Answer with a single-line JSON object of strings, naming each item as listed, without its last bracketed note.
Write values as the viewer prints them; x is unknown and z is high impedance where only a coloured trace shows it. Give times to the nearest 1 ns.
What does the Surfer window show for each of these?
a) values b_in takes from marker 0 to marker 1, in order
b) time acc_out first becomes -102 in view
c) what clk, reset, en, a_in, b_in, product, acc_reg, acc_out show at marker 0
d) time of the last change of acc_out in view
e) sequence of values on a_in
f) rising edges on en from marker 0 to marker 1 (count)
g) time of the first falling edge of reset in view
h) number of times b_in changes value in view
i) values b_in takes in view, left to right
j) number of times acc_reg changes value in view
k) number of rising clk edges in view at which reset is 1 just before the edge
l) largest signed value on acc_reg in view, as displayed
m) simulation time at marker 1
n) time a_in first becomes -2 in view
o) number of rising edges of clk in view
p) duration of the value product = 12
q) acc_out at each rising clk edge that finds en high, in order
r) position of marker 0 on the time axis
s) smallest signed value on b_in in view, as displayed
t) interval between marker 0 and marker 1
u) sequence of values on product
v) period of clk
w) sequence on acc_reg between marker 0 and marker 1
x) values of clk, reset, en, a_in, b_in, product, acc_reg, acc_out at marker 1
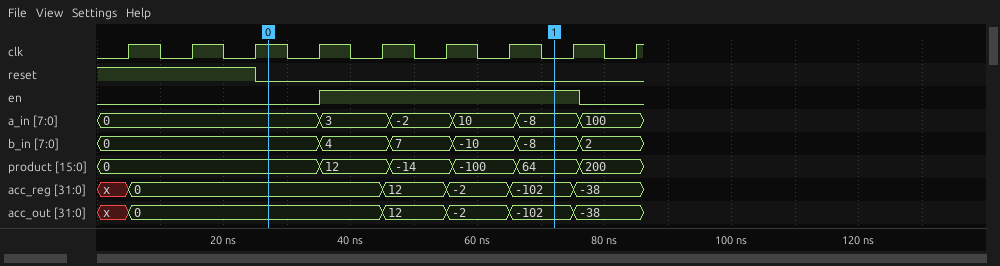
{"values b_in takes from marker 0 to marker 1, in order": "0, 4, 7, -10, -8", "time acc_out first becomes -102 in view": "65 ns", "what clk, reset, en, a_in, b_in, product, acc_reg, acc_out show at marker 0": "clk=1, reset=0, en=0, a_in=0, b_in=0, product=0, acc_reg=0, acc_out=0", "time of the last change of acc_out in view": "75 ns", "sequence of values on a_in": "0, 3, -2, 10, -8, 100", "rising edges on en from marker 0 to marker 1": "1", "time of the first falling edge of reset in view": "25 ns", "number of times b_in changes value in view": "5", "values b_in takes in view, left to right": "0, 4, 7, -10, -8, 2", "number of times acc_reg changes value in view": "5", "number of rising clk edges in view at which reset is 1 just before the edge": "3", "largest signed value on acc_reg in view, as displayed": "12", "simulation time at marker 1": "72 ns", "time a_in first becomes -2 in view": "46 ns", "number of rising edges of clk in view": "9", "duration of the value product = 12": "11 ns", "acc_out at each rising clk edge that finds en high, in order": "0, 12, -2, -102", "position of marker 0 on the time axis": "27 ns", "smallest signed value on b_in in view, as displayed": "-10", "interval between marker 0 and marker 1": "45 ns", "sequence of values on product": "0, 12, -14, -100, 64, 200", "period of clk": "10 ns", "sequence on acc_reg between marker 0 and marker 1": "0, 12, -2, -102", "values of clk, reset, en, a_in, b_in, product, acc_reg, acc_out at marker 1": "clk=0, reset=0, en=1, a_in=-8, b_in=-8, product=64, acc_reg=-102, acc_out=-102"}
